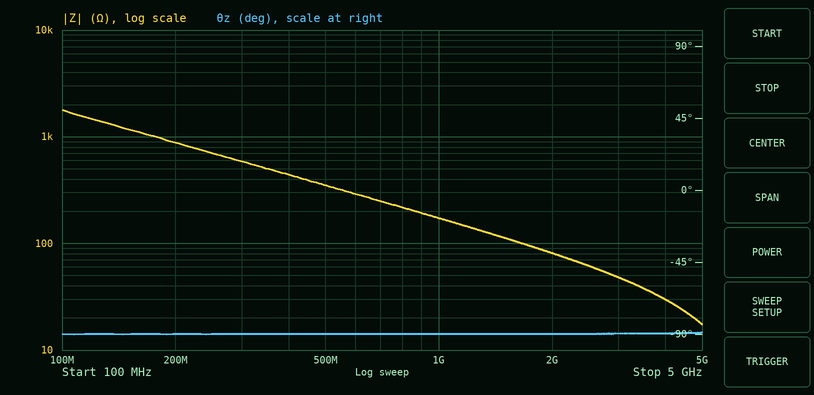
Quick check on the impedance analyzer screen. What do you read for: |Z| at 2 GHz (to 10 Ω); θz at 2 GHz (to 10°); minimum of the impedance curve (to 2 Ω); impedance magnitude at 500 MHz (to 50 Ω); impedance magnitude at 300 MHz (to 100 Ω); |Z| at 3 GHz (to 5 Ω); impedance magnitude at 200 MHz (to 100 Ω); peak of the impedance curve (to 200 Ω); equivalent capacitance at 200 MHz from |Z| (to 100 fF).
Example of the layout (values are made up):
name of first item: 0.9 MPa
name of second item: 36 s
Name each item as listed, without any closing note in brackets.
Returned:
|Z| at 2 GHz: 80 Ω
θz at 2 GHz: -90°
minimum of the impedance curve: 18 Ω
impedance magnitude at 500 MHz: 350 Ω
impedance magnitude at 300 MHz: 600 Ω
|Z| at 3 GHz: 50 Ω
impedance magnitude at 200 MHz: 900 Ω
peak of the impedance curve: 1.8 kΩ
equivalent capacitance at 200 MHz from |Z|: 900 fF
